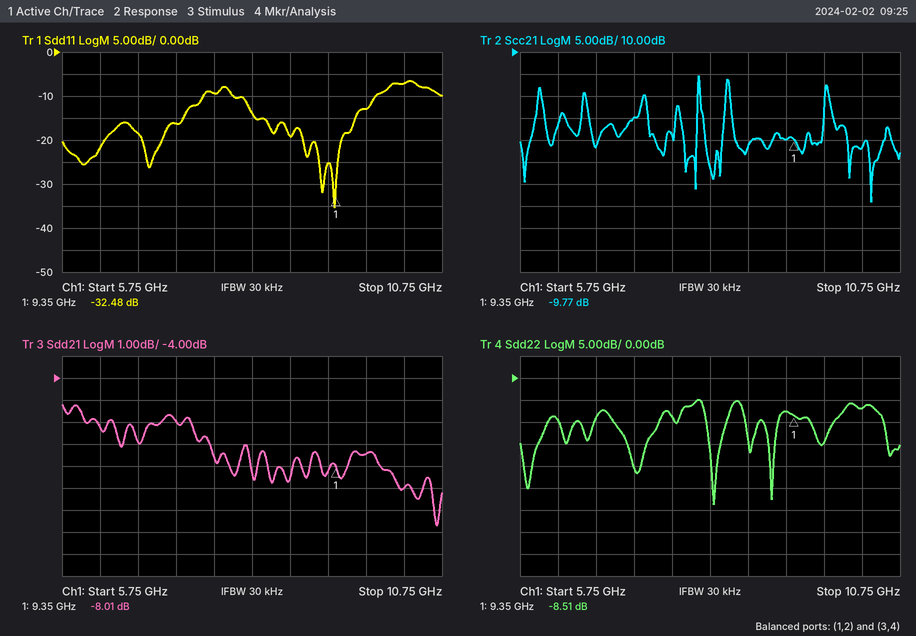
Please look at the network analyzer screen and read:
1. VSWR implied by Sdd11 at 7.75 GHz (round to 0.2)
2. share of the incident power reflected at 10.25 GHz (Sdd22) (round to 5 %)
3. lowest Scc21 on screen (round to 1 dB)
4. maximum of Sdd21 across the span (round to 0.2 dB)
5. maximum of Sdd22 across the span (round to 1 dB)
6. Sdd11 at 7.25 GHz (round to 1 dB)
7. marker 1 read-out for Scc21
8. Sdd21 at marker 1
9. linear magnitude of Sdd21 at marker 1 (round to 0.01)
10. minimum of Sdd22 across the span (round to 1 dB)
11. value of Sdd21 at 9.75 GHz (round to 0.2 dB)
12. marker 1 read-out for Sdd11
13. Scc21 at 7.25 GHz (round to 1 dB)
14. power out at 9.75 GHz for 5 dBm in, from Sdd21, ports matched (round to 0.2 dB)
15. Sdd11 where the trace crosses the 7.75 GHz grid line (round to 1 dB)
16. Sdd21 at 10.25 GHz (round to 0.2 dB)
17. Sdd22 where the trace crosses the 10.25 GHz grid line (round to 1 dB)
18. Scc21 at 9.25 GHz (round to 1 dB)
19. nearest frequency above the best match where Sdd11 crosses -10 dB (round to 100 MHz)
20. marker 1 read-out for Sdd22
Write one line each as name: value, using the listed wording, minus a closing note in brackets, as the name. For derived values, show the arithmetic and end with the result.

VSWR implied by Sdd11 at 7.75 GHz: |Γ| = 10^(-9/20) = 0.3548; VSWR = (1 + 0.3548)/(1 − 0.3548) ≈ 2.10, so 2.0 to the nearest 0.2
share of the incident power reflected at 10.25 GHz (Sdd22): 10^(-7/10) ≈ 20 %
lowest Scc21 on screen: -24 dB
maximum of Sdd21 across the span: -5.2 dB
maximum of Sdd22 across the span: -5 dB
Sdd11 at 7.25 GHz: -16 dB
marker 1 read-out for Scc21: -9.77 dB
Sdd21 at marker 1: -8.01 dB
linear magnitude of Sdd21 at marker 1: 10^(-8.01/20) ≈ 0.40
minimum of Sdd22 across the span: -29 dB
value of Sdd21 at 9.75 GHz: -7.4 dB
marker 1 read-out for Sdd11: -32.48 dB
Scc21 at 7.25 GHz: -5 dB
power out at 9.75 GHz for 5 dBm in, from Sdd21, ports matched: 5 dBm + (-7.4 dB) = -2.4 dBm
Sdd11 where the trace crosses the 7.75 GHz grid line: -9 dB
Sdd21 at 10.25 GHz: -9.0 dB
Sdd22 where the trace crosses the 10.25 GHz grid line: -7 dB
Scc21 at 9.25 GHz: -10 dB
nearest frequency above the best match where Sdd11 crosses -10 dB: 9.9 GHz
marker 1 read-out for Sdd22: -8.51 dB
